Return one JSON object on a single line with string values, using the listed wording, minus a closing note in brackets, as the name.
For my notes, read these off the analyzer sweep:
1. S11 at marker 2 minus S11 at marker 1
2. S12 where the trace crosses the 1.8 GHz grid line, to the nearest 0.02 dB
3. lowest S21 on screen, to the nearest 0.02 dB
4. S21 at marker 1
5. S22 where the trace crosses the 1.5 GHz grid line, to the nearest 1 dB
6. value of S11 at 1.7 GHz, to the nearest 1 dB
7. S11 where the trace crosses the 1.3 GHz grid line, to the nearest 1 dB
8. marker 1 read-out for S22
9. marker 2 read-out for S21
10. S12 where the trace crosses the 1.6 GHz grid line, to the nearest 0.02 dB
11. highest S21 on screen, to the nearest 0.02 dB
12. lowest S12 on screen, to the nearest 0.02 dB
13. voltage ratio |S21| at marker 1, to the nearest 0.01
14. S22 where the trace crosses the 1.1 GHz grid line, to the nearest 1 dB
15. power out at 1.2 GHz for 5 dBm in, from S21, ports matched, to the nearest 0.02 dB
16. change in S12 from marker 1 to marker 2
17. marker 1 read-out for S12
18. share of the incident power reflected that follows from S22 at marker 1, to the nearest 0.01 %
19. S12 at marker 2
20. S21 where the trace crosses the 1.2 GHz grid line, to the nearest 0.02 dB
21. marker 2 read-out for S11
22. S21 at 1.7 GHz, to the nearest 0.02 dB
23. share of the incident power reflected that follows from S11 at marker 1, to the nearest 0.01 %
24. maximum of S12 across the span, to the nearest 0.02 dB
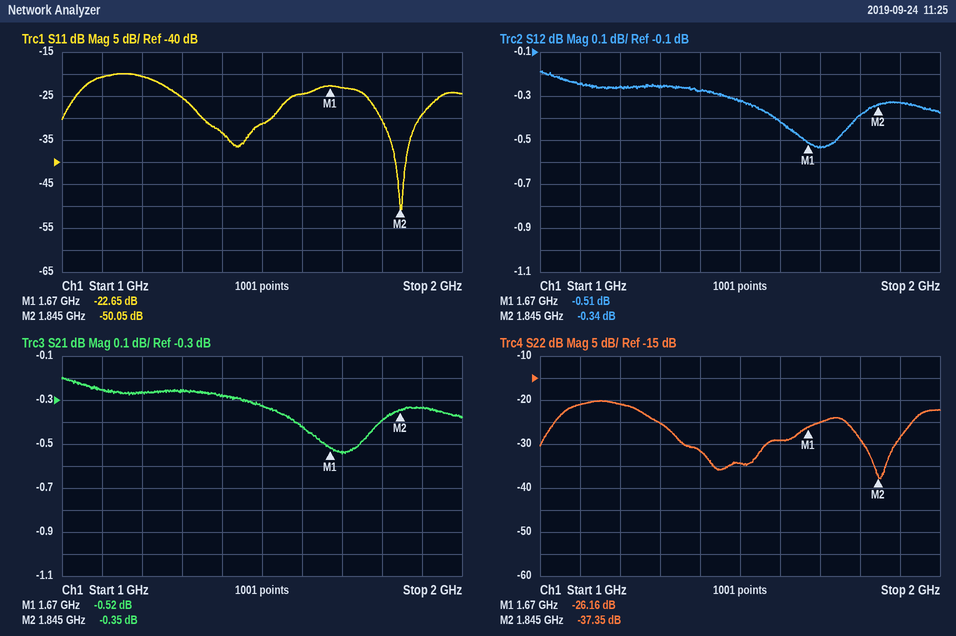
{"S11 at marker 2 minus S11 at marker 1": "-27.40 dB", "S12 where the trace crosses the 1.8 GHz grid line, to the nearest 0.02 dB": "-0.38 dB", "lowest S21 on screen, to the nearest 0.02 dB": "-0.54 dB", "S21 at marker 1": "-0.52 dB", "S22 where the trace crosses the 1.5 GHz grid line, to the nearest 1 dB": "-34 dB", "value of S11 at 1.7 GHz, to the nearest 1 dB": "-23 dB", "S11 where the trace crosses the 1.3 GHz grid line, to the nearest 1 dB": "-25 dB", "marker 1 read-out for S22": "-26.16 dB", "marker 2 read-out for S21": "-0.35 dB", "S12 where the trace crosses the 1.6 GHz grid line, to the nearest 0.02 dB": "-0.42 dB", "highest S21 on screen, to the nearest 0.02 dB": "-0.20 dB", "lowest S12 on screen, to the nearest 0.02 dB": "-0.54 dB", "voltage ratio |S21| at marker 1, to the nearest 0.01": "0.94", "S22 where the trace crosses the 1.1 GHz grid line, to the nearest 1 dB": "-21 dB", "power out at 1.2 GHz for 5 dBm in, from S21, ports matched, to the nearest 0.02 dB": "4.74 dBm", "change in S12 from marker 1 to marker 2": "0.17 dB", "marker 1 read-out for S12": "-0.51 dB", "share of the incident power reflected that follows from S22 at marker 1, to the nearest 0.01 %": "0.24 %", "S12 at marker 2": "-0.34 dB", "S21 where the trace crosses the 1.2 GHz grid line, to the nearest 0.02 dB": "-0.26 dB", "marker 2 read-out for S11": "-50.05 dB", "S21 at 1.7 GHz, to the nearest 0.02 dB": "-0.54 dB", "share of the incident power reflected that follows from S11 at marker 1, to the nearest 0.01 %": "0.54 %", "maximum of S12 across the span, to the nearest 0.02 dB": "-0.18 dB"}
